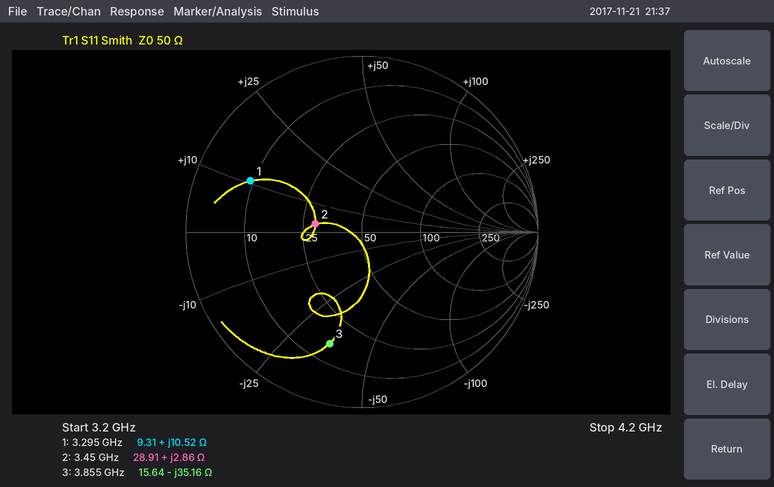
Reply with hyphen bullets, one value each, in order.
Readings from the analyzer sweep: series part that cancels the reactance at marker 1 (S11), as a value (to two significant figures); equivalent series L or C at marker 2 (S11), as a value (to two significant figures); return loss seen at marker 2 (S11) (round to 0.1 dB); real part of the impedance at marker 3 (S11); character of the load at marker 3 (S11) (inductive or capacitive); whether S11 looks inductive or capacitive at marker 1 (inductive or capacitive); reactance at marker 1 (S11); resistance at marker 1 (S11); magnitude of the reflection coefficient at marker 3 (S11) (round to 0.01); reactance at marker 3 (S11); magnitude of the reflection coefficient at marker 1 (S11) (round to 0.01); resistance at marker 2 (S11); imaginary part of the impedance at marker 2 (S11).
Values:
- 4.6 pF
- 130 pH
- 11.4 dB
- 15.64 Ω
- capacitive
- inductive
- +10.52 Ω
- 9.31 Ω
- 0.66
- -35.16 Ω
- 0.70
- 28.91 Ω
- +2.86 Ω
